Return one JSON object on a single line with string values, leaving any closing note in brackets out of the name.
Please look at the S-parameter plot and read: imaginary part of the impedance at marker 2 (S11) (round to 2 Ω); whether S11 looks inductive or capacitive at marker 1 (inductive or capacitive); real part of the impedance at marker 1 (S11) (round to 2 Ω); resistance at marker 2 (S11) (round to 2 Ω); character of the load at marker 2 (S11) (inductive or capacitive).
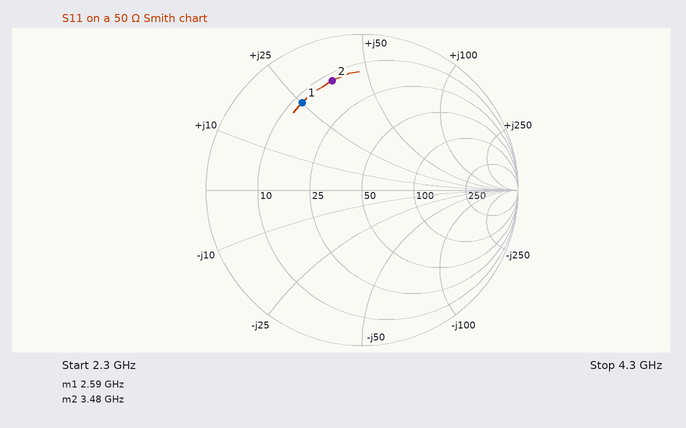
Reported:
{"imaginary part of the impedance at marker 2 (S11)": "+36 Ω", "whether S11 looks inductive or capacitive at marker 1": "inductive", "real part of the impedance at marker 1 (S11)": "12 Ω", "resistance at marker 2 (S11)": "12 Ω", "character of the load at marker 2 (S11)": "inductive"}
